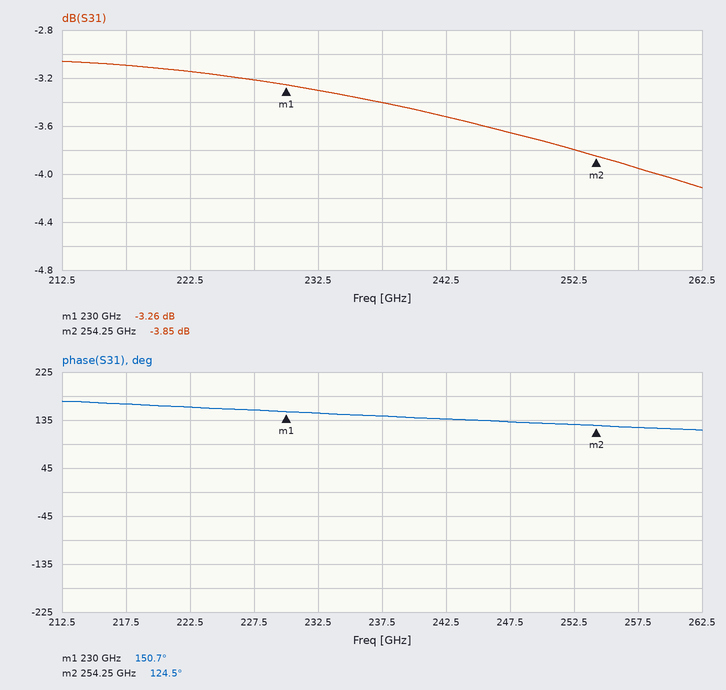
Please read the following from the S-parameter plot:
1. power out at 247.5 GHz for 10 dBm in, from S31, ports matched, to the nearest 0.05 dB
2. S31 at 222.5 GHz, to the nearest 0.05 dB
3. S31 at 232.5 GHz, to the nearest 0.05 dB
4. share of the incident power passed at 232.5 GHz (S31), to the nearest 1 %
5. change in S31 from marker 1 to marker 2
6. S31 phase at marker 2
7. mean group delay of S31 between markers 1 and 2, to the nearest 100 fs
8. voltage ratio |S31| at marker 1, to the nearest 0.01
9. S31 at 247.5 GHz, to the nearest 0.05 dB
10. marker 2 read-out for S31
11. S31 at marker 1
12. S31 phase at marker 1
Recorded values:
6.35 dBm
-3.15 dB
-3.30 dB
47 %
-0.59 dB
124.5°
3.0 ps
0.69
-3.65 dB
-3.85 dB
-3.26 dB
150.7°
